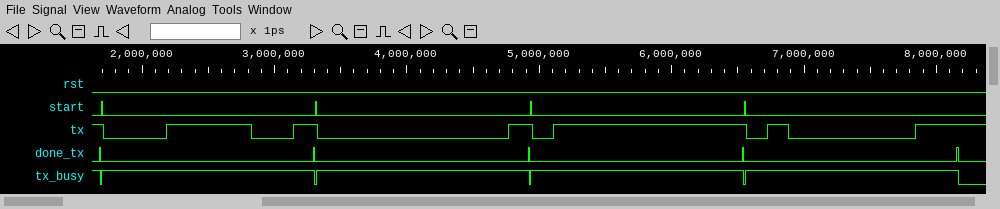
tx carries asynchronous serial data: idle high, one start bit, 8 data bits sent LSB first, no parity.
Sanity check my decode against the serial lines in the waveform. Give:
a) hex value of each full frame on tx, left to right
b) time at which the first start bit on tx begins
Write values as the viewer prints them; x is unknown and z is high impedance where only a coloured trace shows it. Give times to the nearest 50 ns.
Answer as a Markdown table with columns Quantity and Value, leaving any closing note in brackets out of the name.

| Quantity | Value |
|---|---|
| hex value of each full frame on tx, left to right | 3C, 00, FF, 81 |
| time at which the first start bit on tx begins | 1700 ns |
